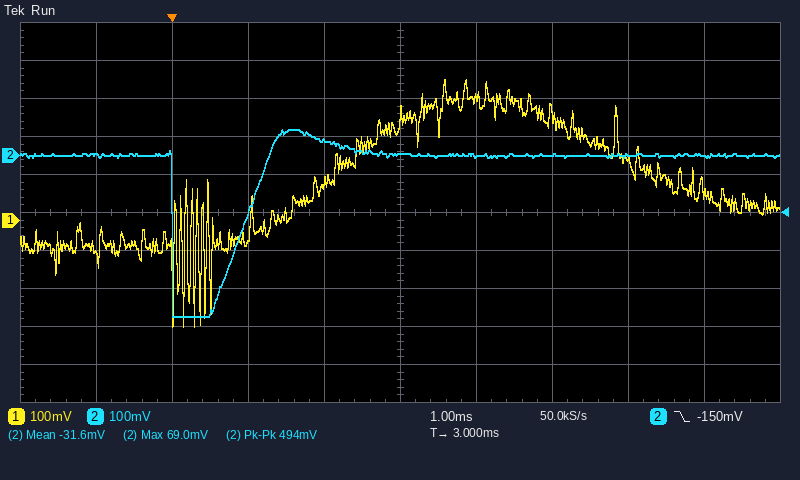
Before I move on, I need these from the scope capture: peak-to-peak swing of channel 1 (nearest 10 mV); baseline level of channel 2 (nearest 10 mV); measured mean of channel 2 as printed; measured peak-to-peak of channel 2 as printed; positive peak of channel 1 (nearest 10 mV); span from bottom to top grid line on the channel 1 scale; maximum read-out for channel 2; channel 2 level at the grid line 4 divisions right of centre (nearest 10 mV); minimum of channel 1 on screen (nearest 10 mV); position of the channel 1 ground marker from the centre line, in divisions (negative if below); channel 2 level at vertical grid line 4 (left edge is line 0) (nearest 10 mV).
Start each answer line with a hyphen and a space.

- 650 mV
- 0 mV
- -31.6 mV
- 494 mV
- 370 mV
- 1 V
- 69.0 mV
- 0 mV
- -280 mV
- -0.2 div
- 40 mV
